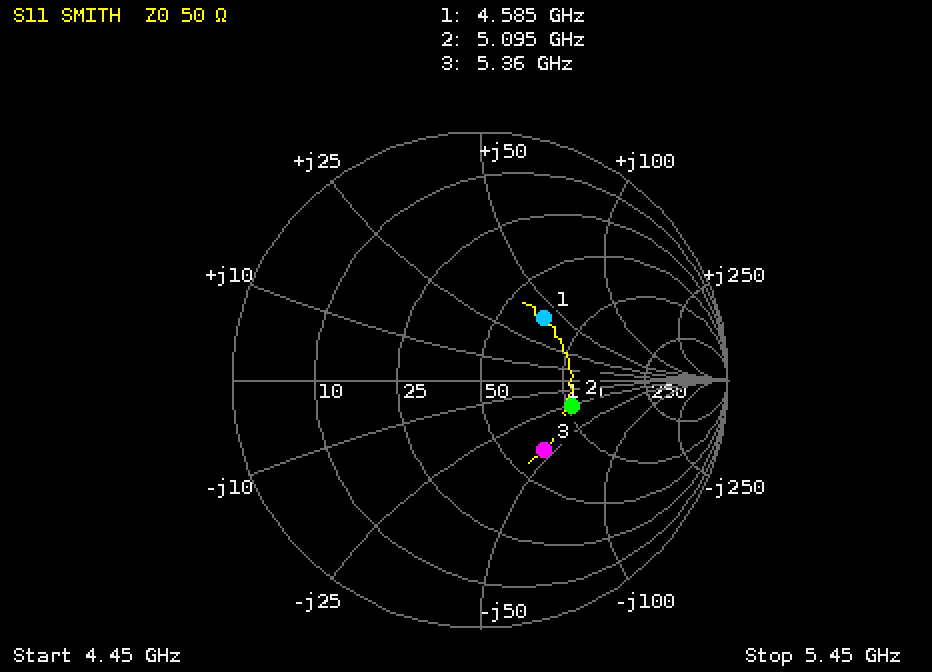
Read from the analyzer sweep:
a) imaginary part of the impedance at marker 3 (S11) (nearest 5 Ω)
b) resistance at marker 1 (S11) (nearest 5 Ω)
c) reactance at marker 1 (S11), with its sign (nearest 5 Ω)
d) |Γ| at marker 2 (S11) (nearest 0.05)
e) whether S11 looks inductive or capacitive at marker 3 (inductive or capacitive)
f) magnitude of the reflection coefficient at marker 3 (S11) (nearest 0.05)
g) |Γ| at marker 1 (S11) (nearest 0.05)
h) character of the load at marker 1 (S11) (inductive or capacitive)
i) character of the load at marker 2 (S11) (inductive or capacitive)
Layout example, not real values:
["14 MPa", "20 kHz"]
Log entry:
["-45 Ω", "70 Ω", "+40 Ω", "0.40", "capacitive", "0.40", "0.35", "inductive", "capacitive"]
